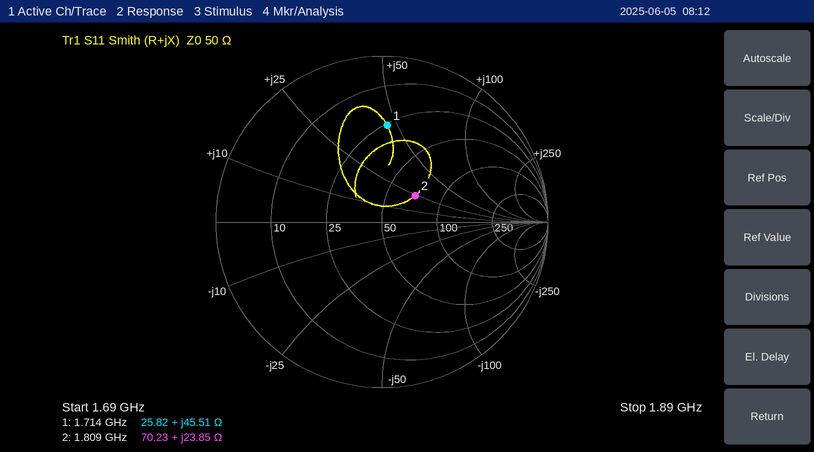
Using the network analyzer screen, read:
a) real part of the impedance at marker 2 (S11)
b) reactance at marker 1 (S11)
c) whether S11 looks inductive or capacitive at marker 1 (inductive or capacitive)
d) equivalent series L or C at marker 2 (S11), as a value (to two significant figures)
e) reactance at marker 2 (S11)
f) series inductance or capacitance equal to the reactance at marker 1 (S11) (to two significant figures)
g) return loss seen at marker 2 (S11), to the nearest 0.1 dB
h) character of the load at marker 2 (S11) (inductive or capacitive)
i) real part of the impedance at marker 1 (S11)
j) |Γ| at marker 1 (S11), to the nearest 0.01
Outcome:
70.23 Ω
+45.51 Ω
inductive
2.1 nH
+23.85 Ω
4.2 nH
11.9 dB
inductive
25.82 Ω
0.58
